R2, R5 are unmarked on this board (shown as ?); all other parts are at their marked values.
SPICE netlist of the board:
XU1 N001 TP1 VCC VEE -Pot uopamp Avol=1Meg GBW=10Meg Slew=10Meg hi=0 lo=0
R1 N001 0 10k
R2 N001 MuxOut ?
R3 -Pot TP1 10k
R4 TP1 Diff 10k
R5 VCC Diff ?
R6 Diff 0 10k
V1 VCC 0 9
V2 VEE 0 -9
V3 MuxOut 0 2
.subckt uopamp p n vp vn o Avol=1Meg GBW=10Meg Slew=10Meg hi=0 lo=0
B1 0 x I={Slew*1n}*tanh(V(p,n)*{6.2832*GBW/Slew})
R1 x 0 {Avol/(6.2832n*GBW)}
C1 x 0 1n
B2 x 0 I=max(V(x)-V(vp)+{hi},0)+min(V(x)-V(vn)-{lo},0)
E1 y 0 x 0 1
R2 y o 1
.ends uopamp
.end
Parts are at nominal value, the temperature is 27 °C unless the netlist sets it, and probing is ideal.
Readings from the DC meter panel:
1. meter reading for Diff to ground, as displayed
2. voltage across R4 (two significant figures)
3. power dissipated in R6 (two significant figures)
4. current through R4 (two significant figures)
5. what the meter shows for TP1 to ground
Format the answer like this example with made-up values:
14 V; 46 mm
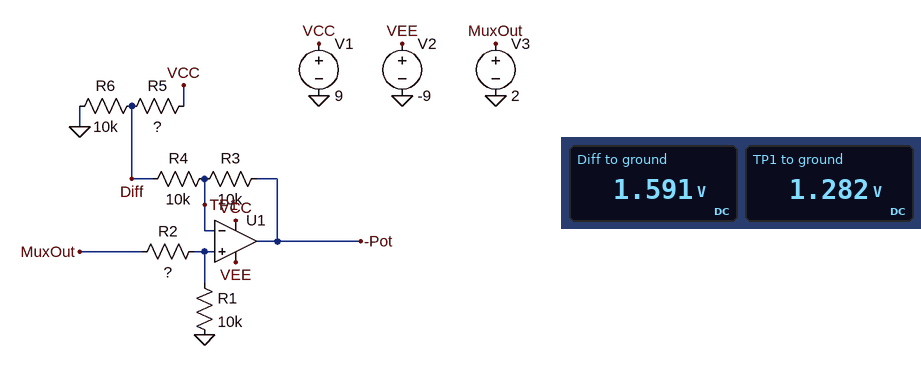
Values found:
1.591 V; 310 mV; 250 µW; 31 µA; 1.282 V
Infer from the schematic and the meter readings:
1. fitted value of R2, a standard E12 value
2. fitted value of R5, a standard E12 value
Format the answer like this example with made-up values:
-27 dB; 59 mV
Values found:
5.6 kΩ; 39 kΩ
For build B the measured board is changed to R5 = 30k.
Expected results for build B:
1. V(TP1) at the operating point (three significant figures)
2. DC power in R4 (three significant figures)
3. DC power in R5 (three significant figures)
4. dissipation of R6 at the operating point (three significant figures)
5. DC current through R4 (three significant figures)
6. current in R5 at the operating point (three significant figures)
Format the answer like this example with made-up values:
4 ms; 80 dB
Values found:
1.28 V; 30.6 µW; 1.71 mW; 337 µW; 55.3 µA; 239 µA
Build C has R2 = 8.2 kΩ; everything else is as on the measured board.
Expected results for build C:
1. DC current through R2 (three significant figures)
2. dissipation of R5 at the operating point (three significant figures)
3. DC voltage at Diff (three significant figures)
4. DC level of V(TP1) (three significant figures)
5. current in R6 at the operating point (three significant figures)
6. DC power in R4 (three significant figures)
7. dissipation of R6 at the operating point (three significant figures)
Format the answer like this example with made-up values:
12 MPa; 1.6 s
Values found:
110 µA; 1.44 mW; 1.51 V; 1.10 V; 151 µA; 16.9 µW; 228 µW
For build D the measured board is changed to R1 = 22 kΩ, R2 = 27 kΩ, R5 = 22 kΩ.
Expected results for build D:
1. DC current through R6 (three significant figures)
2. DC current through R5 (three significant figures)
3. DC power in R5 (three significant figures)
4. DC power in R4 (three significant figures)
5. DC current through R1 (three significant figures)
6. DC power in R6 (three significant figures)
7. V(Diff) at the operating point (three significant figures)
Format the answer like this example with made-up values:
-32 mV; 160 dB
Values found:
203 µA; 317 µA; 2.21 mW; 129 µW; 40.8 µA; 413 µW; 2.03 V
